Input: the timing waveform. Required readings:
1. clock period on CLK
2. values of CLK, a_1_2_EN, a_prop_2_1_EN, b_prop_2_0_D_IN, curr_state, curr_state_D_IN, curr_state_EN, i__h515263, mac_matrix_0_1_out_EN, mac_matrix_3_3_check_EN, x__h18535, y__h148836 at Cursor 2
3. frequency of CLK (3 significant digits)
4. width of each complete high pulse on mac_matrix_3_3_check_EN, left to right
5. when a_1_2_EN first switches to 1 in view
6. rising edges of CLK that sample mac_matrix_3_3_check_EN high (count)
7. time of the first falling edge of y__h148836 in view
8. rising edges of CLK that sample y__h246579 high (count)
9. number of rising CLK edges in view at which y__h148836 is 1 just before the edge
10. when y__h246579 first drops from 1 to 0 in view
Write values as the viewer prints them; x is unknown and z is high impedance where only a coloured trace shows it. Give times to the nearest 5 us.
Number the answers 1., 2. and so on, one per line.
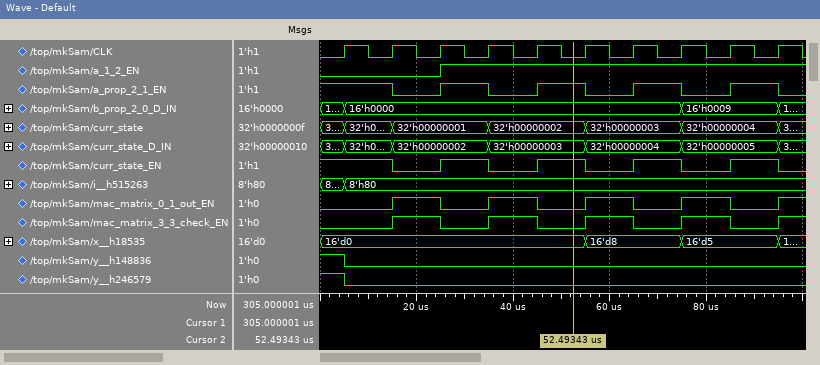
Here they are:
1. 10 us
2. CLK=0, a_1_2_EN=1, a_prop_2_1_EN=1, b_prop_2_0_D_IN=16'h0000, curr_state=32'h00000002, curr_state_D_IN=32'h00000003, curr_state_EN=1, i__h515263=8'h80, mac_matrix_0_1_out_EN=0, mac_matrix_3_3_check_EN=0, x__h18535=16'd0, y__h148836=0
3. 100 kHz
4. 10 us, 10 us, 10 us, 10 us
5. 25 us
6. 4
7. 5 us
8. 1
9. 1
10. 5 us
